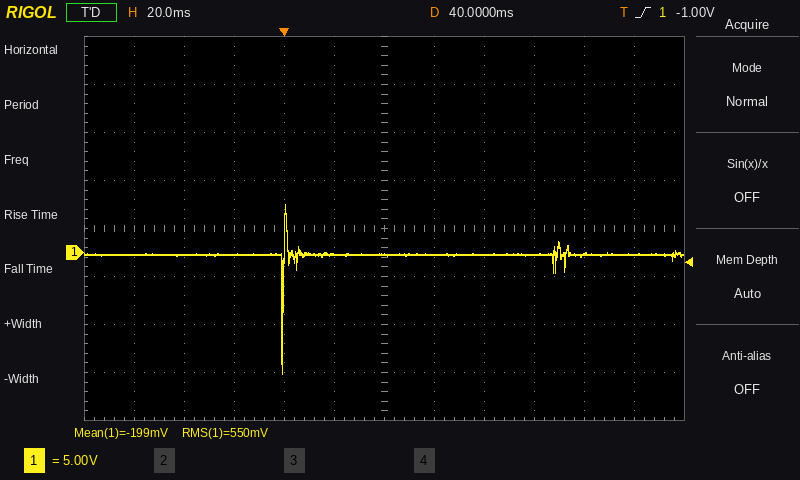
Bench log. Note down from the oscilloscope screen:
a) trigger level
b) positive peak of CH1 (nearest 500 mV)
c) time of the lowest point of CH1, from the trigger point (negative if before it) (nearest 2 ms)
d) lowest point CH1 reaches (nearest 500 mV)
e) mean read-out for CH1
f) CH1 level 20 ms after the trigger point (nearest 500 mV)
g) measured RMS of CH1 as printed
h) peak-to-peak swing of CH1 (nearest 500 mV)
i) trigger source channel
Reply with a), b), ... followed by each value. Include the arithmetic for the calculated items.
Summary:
a) -1.00 V
b) 5.0 V
c) 0 ms
d) -12.5 V
e) -199 mV
f) 0.0 V
g) 550 mV
h) 5.0 V − (-12.5 V) = 17.5 V
i) CH1
